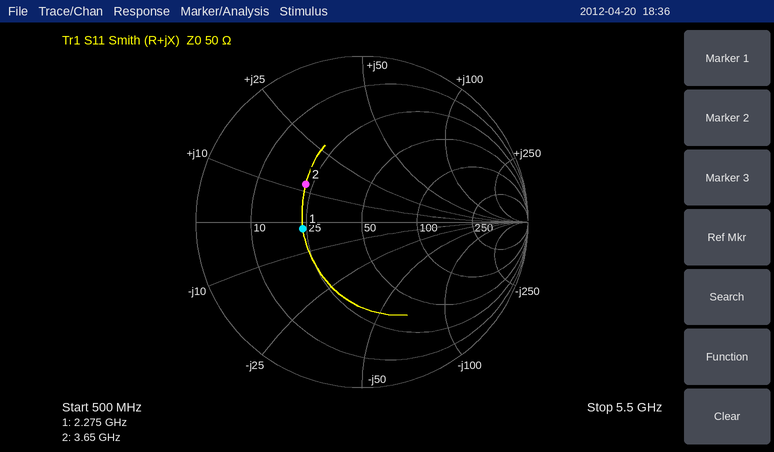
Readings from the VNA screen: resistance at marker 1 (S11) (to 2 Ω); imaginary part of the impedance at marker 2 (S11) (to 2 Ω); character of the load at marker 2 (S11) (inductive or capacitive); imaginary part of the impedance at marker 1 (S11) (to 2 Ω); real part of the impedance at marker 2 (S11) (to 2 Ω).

24 Ω
+12 Ω
inductive
-2 Ω
22 Ω
